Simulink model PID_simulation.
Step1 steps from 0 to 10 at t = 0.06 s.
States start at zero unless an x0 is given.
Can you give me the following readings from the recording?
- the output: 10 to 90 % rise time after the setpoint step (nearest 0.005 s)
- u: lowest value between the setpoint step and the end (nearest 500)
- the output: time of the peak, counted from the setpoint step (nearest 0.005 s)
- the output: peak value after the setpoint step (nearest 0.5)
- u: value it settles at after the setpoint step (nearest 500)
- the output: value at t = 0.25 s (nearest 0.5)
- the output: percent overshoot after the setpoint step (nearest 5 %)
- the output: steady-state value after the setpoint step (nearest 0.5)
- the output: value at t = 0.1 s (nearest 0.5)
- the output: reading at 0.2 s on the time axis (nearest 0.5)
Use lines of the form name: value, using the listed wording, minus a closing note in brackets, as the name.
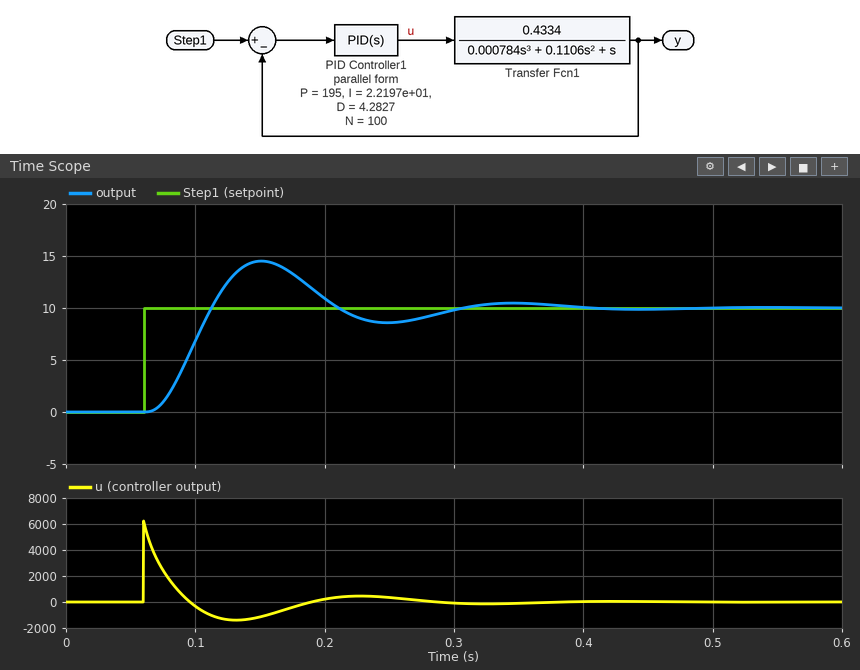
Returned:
the output: 10 to 90 % rise time after the setpoint step: 0.035 s
u: lowest value between the setpoint step and the end: -1500
the output: time of the peak, counted from the setpoint step: 0.090 s
the output: peak value after the setpoint step: 14.5
u: value it settles at after the setpoint step: 0
the output: value at t = 0.25 s: 8.5
the output: percent overshoot after the setpoint step: 45 %
the output: steady-state value after the setpoint step: 10.0
the output: value at t = 0.1 s: 7.0
the output: reading at 0.2 s on the time axis: 11.0
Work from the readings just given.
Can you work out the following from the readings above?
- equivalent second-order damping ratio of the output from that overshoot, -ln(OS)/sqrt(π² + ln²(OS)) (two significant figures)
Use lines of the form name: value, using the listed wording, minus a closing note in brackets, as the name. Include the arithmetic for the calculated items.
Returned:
equivalent second-order damping ratio of the output from that overshoot, -ln(OS)/sqrt(π² + ln²(OS)): ln(0.45) = -0.799; 0.799 / sqrt(9.870 + 0.638) = 0.25
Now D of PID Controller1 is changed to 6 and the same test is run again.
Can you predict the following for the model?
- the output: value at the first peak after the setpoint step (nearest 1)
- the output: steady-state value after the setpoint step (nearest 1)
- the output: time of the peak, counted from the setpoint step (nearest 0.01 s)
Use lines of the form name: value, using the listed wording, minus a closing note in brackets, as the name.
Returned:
the output: value at the first peak after the setpoint step: 14
the output: steady-state value after the setpoint step: 10
the output: time of the peak, counted from the setpoint step: 0.08 s
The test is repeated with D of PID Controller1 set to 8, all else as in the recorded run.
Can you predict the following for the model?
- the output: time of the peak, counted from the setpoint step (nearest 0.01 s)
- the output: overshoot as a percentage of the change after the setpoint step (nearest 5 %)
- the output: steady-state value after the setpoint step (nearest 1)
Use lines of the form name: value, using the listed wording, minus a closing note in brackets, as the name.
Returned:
the output: time of the peak, counted from the setpoint step: 0.07 s
the output: overshoot as a percentage of the change after the setpoint step: 35 %
the output: steady-state value after the setpoint step: 10
